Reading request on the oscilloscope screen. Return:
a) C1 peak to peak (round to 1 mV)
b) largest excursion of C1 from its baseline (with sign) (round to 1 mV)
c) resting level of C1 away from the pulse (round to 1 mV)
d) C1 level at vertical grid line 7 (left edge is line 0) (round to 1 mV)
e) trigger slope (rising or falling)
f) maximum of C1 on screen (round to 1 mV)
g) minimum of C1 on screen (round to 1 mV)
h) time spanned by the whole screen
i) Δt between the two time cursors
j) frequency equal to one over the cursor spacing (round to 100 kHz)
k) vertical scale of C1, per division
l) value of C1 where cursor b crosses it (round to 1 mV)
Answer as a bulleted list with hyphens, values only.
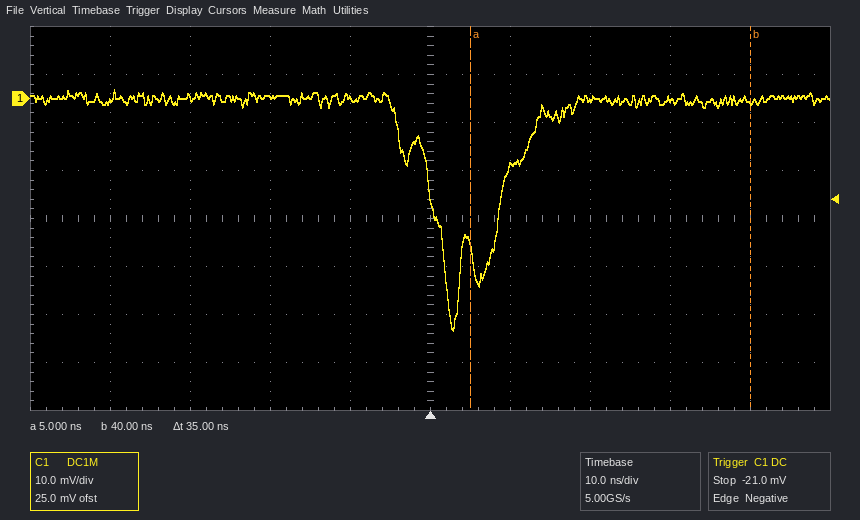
- 50 mV
- -48 mV
- 0 mV
- 0 mV
- falling
- 2 mV
- -48 mV
- 100 ns
- 35 ns
- 28.6 MHz
- 10 mV
- -1 mV
